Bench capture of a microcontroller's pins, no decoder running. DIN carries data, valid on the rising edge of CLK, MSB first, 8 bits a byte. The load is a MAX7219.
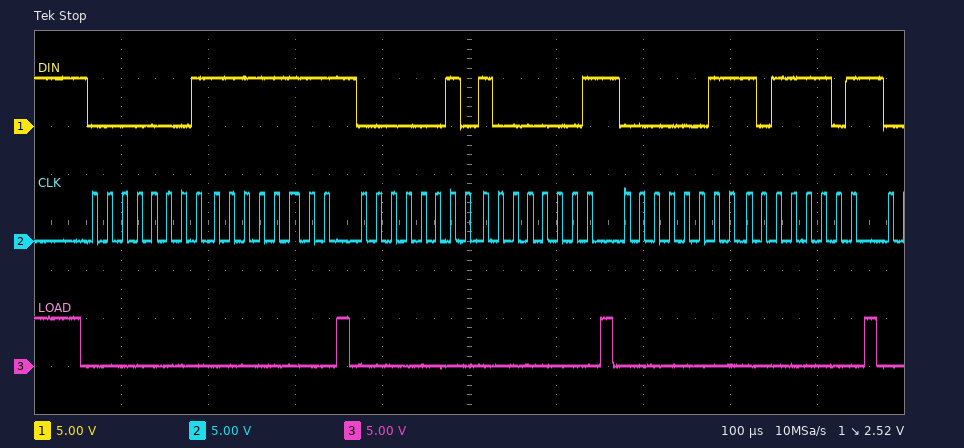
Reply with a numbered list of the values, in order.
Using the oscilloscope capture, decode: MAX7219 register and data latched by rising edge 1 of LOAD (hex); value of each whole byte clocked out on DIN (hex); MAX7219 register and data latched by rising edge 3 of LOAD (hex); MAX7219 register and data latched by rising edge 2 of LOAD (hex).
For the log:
1. register 0x1, data 0xFF
2. 0x01 0xFF 0x02 0x81 0x03 0xBD
3. register 0x3, data 0xBD
4. register 0x2, data 0x81
